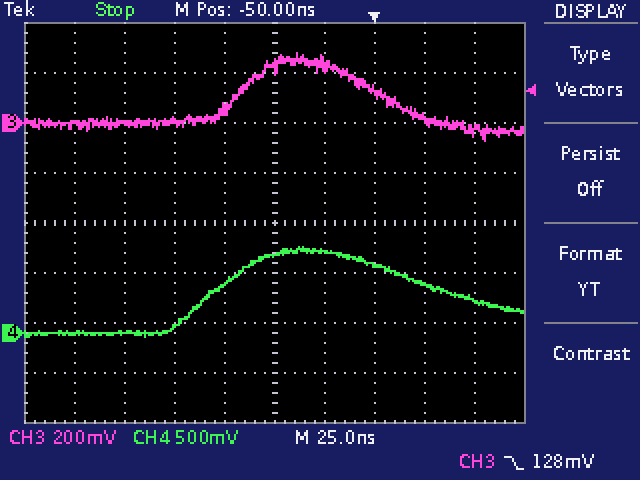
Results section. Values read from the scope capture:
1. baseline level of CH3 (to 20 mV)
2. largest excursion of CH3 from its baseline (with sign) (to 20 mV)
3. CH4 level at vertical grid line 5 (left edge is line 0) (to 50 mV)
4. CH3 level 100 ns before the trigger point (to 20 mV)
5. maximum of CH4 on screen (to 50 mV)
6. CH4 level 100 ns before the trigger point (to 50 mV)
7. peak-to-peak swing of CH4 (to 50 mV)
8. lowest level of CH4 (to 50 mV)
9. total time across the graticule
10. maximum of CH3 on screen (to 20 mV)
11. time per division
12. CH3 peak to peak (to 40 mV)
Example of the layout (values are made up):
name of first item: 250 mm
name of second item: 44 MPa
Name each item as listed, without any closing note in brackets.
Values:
baseline level of CH3: 0 mV
largest excursion of CH3 from its baseline (with sign): +280 mV
CH4 level at vertical grid line 5 (left edge is line 0): 800 mV
CH3 level 100 ns before the trigger point: 0 mV
maximum of CH4 on screen: 850 mV
CH4 level 100 ns before the trigger point: 50 mV
peak-to-peak swing of CH4: 900 mV
lowest level of CH4: -50 mV
total time across the graticule: 250 ns
maximum of CH3 on screen: 280 mV
time per division: 25 ns
CH3 peak to peak: 360 mV
